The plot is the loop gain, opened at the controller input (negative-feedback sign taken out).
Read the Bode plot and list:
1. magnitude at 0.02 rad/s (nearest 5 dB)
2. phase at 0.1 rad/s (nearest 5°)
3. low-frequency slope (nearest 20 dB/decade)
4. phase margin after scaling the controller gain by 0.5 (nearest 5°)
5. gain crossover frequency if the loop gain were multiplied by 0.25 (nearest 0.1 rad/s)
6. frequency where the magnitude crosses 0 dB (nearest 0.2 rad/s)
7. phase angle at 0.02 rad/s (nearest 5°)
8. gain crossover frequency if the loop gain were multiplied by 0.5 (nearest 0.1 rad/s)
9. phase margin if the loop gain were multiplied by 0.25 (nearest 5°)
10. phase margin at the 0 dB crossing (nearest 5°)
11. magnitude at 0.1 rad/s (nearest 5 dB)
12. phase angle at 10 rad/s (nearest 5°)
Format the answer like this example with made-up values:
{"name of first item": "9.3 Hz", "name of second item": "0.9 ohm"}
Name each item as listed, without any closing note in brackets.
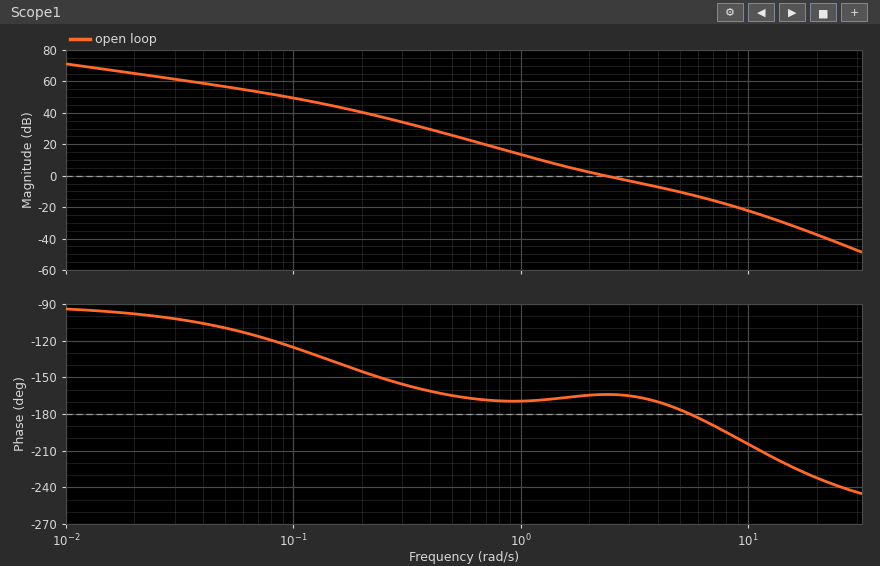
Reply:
{"magnitude at 0.02 rad/s": "65 dB", "phase at 0.1 rad/s": "-125°", "low-frequency slope": "-20 dB/decade", "phase margin after scaling the controller gain by 0.5": "15°", "gain crossover frequency if the loop gain were multiplied by 0.25": "1.1 rad/s", "frequency where the magnitude crosses 0 dB": "2.4 rad/s", "phase angle at 0.02 rad/s": "-100°", "gain crossover frequency if the loop gain were multiplied by 0.5": "1.6 rad/s", "phase margin if the loop gain were multiplied by 0.25": "10°", "phase margin at the 0 dB crossing": "15°", "magnitude at 0.1 rad/s": "50 dB", "phase angle at 10 rad/s": "-205°"}
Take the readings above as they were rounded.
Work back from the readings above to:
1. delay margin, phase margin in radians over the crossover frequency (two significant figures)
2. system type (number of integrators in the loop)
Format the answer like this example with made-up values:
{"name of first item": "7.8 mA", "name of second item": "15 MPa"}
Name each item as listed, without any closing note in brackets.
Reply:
{"delay margin, phase margin in radians over the crossover frequency": "0.11 s", "system type": "1"}
